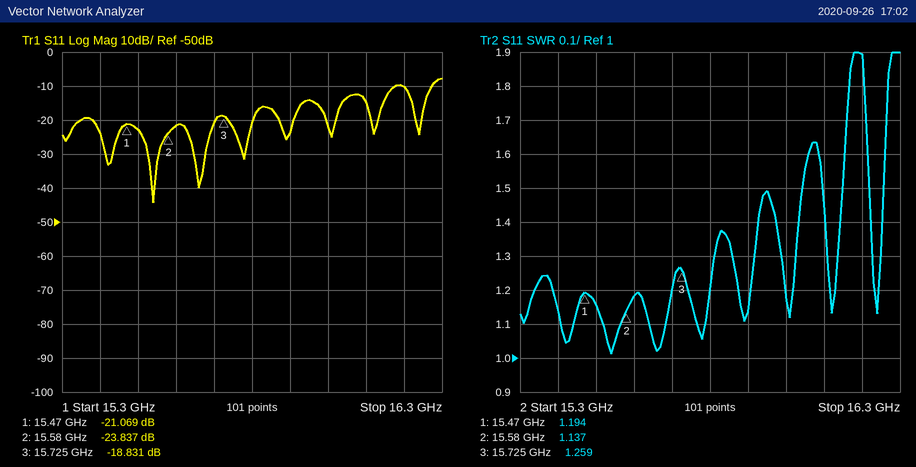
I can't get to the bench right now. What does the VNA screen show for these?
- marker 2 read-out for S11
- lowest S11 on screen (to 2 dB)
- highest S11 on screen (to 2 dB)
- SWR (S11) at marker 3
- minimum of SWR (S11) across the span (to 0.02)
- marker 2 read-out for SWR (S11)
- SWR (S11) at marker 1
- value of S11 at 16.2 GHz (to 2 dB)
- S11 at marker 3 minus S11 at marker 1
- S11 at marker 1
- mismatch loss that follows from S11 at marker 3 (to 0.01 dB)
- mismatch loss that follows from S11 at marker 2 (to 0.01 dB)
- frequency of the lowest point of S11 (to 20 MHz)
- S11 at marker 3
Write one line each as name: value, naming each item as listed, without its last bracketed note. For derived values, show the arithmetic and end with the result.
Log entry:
marker 2 read-out for S11: -23.837 dB
lowest S11 on screen: -44 dB
highest S11 on screen: -8 dB
SWR (S11) at marker 3: 1.259
minimum of SWR (S11) across the span: 1.02
marker 2 read-out for SWR: 1.137
SWR (S11) at marker 1: 1.194
value of S11 at 16.2 GHz: -10 dB
S11 at marker 3 minus S11 at marker 1: -18.831 − (-21.069) = 2.238 dB
S11 at marker 1: -21.069 dB
mismatch loss that follows from S11 at marker 3: −10 log10(1 − 10^(-18.831/10)) ≈ 0.06 dB
mismatch loss that follows from S11 at marker 2: −10 log10(1 − 10^(-23.837/10)) ≈ 0.02 dB
frequency of the lowest point of S11: 15.54 GHz
S11 at marker 3: -18.831 dB
